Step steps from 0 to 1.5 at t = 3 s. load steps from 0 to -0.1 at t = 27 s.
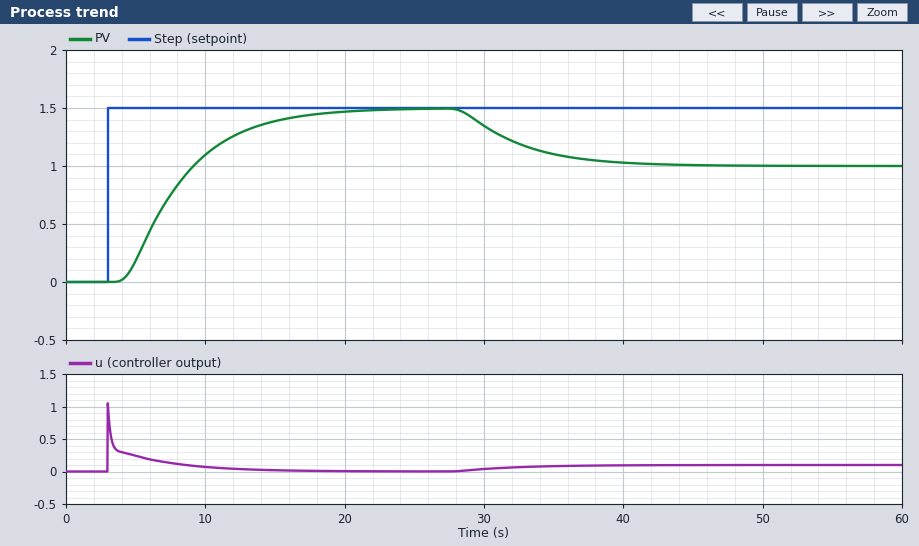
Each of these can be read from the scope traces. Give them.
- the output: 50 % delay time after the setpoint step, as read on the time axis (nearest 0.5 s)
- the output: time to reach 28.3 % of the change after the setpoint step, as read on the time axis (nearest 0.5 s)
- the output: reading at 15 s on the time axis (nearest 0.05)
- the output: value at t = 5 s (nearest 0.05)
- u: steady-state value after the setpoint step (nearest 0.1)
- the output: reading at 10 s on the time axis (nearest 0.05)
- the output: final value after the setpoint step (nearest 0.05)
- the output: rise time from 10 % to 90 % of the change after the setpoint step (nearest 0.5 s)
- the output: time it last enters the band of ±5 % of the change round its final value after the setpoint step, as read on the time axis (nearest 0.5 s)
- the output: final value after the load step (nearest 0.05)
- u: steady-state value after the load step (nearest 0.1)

7.5 s
6.0 s
1.40
0.20
0.0
1.10
1.50
9.0 s
16.5 s
1.00
0.1
